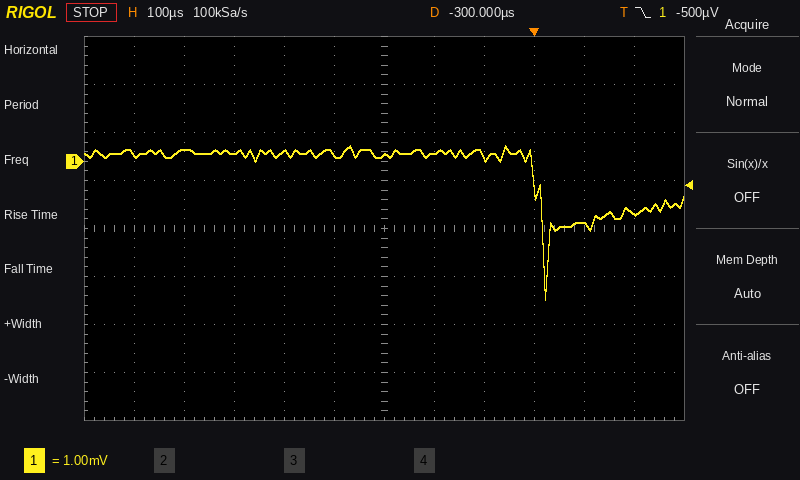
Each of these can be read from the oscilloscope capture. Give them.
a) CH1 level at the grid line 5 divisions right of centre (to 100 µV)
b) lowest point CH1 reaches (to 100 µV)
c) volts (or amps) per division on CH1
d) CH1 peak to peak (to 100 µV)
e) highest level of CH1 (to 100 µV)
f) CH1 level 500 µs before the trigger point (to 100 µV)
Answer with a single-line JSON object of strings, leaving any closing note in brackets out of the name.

{"CH1 level at the grid line 5 divisions right of centre": "-1.1 mV", "lowest point CH1 reaches": "-2.9 mV", "volts (or amps) per division on CH1": "1 mV", "CH1 peak to peak": "3.2 mV", "highest level of CH1": "300 µV", "CH1 level 500 µs before the trigger point": "200 µV"}
